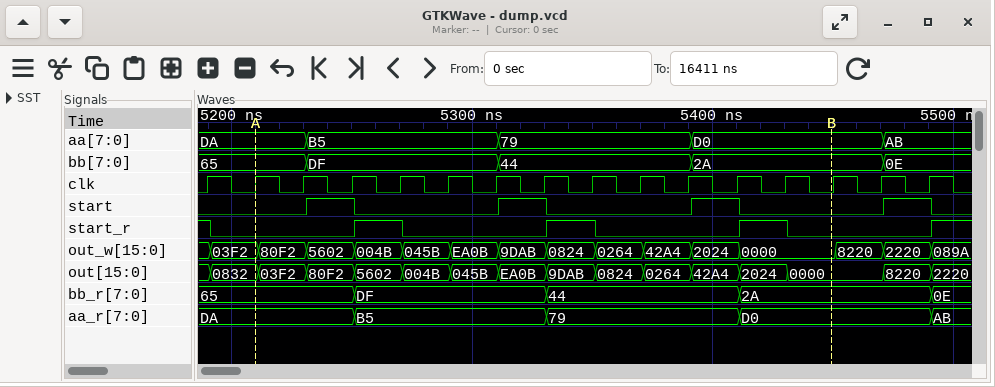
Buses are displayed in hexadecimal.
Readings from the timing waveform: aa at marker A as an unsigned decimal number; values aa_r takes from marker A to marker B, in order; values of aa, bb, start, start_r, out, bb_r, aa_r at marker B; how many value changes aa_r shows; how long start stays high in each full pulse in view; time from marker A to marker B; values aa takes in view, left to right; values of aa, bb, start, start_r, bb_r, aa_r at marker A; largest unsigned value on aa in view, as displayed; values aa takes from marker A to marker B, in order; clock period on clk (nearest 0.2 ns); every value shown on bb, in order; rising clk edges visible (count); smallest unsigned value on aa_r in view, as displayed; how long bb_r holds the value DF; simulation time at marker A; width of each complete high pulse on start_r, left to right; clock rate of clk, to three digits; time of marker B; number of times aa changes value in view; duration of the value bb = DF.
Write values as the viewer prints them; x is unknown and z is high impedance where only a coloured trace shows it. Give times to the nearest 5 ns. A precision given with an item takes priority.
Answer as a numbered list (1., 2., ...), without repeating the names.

1. 218
2. DA, B5, 79, D0
3. aa=D0, bb=2A, start=0, start_r=0, out=0000, bb_r=2A, aa_r=D0
4. 4
5. 20 ns, 20 ns, 20 ns, 20 ns
6. 240 ns
7. DA, B5, 79, D0, AB
8. aa=DA, bb=65, start=0, start_r=0, bb_r=65, aa_r=DA
9. DA
10. DA, B5, 79, D0
11. 20 ns
12. 65, DF, 44, 2A, 0E
13. 16
14. 79
15. 80 ns
16. 5210 ns
17. 20 ns, 20 ns, 20 ns
18. 50.0 MHz
19. 5450 ns
20. 4
21. 80 ns
